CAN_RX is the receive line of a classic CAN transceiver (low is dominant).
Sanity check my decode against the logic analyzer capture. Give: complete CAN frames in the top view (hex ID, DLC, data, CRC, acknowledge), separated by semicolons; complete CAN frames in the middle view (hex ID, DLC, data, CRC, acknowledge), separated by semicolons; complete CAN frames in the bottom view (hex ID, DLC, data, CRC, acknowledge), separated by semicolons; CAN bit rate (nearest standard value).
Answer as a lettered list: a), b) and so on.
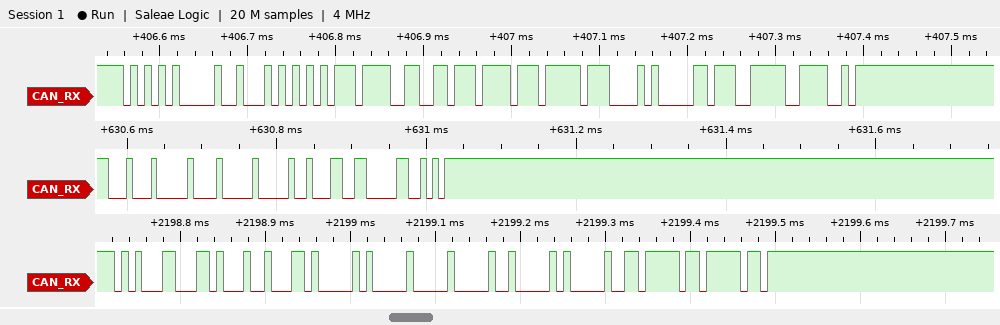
a) ID 550, DLC 8, data AA BB CC DD EE FF 0A 0B, CRC 4FBC, ACK
b) ID 110, DLC 2, data 00 11, CRC 4C12, ACK
c) ID 14611234, DLC 4, data 00 01 02 03, CRC 3FBF, ACK
d) 125 kbit/s
